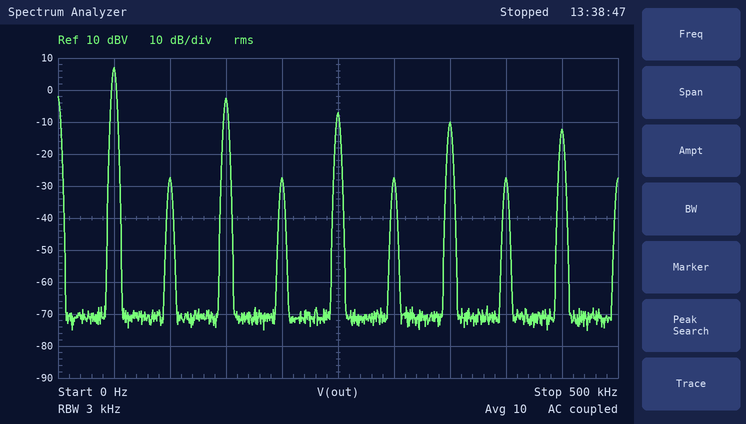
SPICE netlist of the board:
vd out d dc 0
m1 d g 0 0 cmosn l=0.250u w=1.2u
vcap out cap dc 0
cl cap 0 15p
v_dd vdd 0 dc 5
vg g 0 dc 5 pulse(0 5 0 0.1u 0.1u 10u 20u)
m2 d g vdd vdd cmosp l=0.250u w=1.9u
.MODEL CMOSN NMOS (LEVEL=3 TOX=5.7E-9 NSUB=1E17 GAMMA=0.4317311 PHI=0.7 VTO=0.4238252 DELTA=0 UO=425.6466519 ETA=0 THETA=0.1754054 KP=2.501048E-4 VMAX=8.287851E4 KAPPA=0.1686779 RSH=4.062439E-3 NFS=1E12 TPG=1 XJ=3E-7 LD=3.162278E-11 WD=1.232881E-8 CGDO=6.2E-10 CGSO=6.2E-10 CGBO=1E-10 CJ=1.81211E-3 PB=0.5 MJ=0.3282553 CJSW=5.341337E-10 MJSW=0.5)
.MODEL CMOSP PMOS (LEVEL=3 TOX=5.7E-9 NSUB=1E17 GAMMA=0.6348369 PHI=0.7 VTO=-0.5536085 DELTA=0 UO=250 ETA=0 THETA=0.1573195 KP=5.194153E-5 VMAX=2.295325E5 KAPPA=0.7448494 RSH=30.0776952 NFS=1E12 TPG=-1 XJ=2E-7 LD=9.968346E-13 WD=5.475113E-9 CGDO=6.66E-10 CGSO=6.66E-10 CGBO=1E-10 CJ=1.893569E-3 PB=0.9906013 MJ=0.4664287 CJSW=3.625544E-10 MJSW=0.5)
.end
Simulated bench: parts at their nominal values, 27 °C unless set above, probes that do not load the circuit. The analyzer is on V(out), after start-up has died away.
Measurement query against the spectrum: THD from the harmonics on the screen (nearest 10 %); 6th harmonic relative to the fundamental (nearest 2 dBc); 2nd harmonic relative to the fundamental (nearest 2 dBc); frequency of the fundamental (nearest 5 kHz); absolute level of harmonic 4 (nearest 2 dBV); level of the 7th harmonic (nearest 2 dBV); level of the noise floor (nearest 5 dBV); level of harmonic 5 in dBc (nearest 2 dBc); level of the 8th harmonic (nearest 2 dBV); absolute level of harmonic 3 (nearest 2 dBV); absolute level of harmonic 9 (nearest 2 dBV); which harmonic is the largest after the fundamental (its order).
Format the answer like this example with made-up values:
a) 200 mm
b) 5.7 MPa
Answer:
a) 40 %
b) -34 dBc
c) -34 dBc
d) 50 kHz
e) -28 dBV
f) -10 dBV
g) -70 dBV
h) -14 dBc
i) -28 dBV
j) -2 dBV
k) -12 dBV
l) 3
